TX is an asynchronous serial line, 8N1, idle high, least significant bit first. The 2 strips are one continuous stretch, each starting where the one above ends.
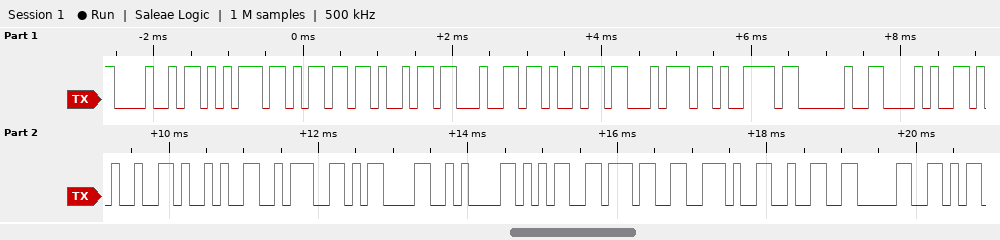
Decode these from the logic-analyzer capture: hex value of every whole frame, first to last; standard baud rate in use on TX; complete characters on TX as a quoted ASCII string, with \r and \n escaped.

48 75 6D 69 64 69 74 79 20 28 25 29 3A 0D 0A 35 37 2E 32 30
9600 baud
"Humidity (%):\r\n57.20"
